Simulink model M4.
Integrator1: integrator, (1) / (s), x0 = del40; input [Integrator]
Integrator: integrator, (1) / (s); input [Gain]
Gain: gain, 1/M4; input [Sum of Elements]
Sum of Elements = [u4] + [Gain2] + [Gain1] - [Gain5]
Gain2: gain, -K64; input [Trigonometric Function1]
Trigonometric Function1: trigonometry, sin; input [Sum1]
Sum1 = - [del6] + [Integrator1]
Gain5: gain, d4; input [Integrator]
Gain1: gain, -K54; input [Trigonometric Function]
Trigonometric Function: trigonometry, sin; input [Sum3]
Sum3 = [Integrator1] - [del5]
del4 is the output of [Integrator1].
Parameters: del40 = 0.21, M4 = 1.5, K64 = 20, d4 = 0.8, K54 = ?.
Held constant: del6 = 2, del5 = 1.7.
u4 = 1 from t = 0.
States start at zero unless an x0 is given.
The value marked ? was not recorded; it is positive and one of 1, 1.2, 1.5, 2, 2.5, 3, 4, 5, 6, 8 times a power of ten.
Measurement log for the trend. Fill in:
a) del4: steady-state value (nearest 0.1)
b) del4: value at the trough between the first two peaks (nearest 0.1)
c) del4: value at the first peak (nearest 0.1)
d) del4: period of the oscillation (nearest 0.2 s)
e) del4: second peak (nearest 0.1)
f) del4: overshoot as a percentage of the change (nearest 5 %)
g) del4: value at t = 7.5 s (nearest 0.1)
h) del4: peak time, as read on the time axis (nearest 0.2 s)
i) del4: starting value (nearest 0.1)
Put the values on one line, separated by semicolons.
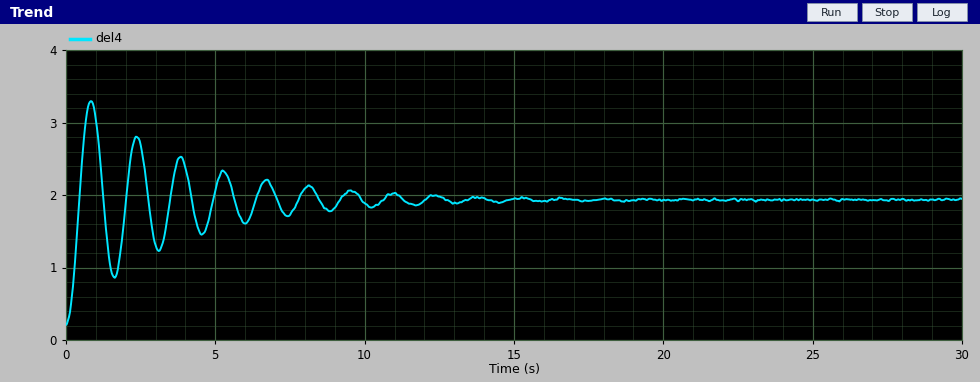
1.9; 0.9; 3.3; 1.6 s; 2.8; 80 %; 1.7; 0.8 s; 0.2
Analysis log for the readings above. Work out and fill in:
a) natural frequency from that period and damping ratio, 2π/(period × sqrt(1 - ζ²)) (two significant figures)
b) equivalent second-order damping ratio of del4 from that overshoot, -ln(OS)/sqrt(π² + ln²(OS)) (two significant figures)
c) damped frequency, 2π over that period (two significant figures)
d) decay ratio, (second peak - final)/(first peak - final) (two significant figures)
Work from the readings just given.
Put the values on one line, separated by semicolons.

3.9 rad/s; 0.071; 3.9 rad/s; 0.64
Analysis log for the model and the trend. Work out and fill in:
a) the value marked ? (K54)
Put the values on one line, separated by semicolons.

10
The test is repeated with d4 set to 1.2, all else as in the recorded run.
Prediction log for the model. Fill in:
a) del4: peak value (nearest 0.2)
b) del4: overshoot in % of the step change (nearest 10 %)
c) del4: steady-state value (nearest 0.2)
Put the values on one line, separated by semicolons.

3.2; 70 %; 2.0
